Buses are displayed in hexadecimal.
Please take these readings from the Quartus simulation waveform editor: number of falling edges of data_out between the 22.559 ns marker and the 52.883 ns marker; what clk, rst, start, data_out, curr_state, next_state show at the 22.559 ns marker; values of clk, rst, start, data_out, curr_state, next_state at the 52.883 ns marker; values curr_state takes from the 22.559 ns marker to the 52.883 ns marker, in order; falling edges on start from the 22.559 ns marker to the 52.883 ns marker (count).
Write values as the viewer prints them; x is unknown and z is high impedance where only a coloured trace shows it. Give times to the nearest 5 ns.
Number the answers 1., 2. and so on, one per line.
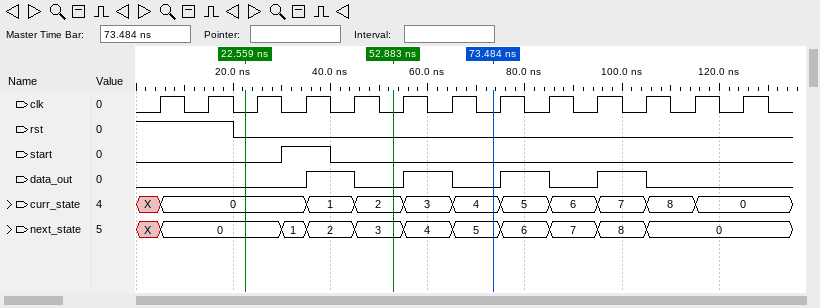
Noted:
1. 1
2. clk=0, rst=0, start=0, data_out=0, curr_state=0, next_state=0
3. clk=0, rst=0, start=0, data_out=0, curr_state=2, next_state=3
4. 0, 1, 2
5. 1
